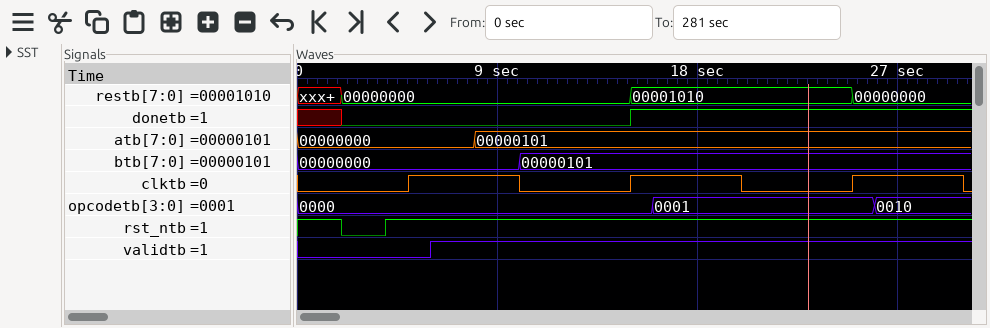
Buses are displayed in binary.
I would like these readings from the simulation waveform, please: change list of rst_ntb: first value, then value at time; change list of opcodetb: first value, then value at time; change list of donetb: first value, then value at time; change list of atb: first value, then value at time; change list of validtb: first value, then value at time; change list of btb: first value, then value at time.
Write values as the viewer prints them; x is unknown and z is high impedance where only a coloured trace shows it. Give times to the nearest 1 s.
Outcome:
1, 0 at 2 s, 1 at 4 s
0000, 0001 at 16 s, 0010 at 26 s
x, 0 at 2 s, 1 at 15 s
00000000, 00000101 at 8 s
0, 1 at 6 s
00000000, 00000101 at 10 s
